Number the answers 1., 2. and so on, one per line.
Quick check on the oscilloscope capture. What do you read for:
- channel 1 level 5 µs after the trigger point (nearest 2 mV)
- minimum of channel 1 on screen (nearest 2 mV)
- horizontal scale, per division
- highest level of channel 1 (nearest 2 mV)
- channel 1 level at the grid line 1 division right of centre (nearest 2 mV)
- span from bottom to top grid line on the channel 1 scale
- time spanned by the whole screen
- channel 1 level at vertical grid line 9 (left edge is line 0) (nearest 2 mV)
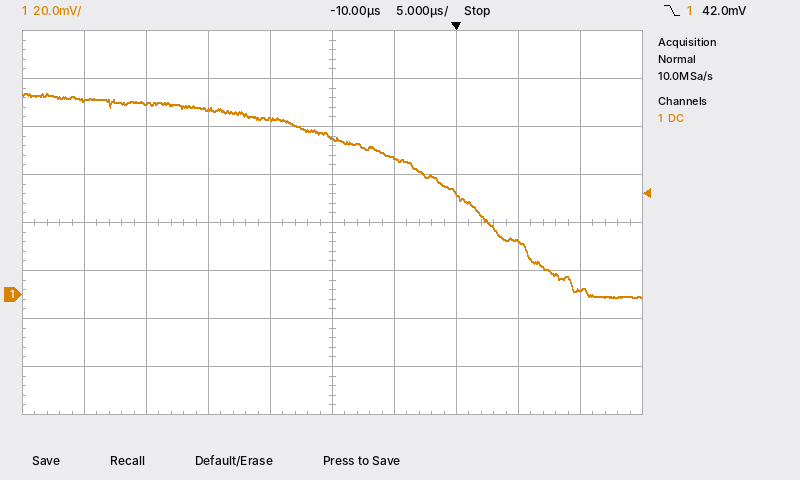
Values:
1. 22 mV
2. -2 mV
3. 5 µs
4. 84 mV
5. 56 mV
6. 160 mV
7. 50 µs
8. 2 mV
